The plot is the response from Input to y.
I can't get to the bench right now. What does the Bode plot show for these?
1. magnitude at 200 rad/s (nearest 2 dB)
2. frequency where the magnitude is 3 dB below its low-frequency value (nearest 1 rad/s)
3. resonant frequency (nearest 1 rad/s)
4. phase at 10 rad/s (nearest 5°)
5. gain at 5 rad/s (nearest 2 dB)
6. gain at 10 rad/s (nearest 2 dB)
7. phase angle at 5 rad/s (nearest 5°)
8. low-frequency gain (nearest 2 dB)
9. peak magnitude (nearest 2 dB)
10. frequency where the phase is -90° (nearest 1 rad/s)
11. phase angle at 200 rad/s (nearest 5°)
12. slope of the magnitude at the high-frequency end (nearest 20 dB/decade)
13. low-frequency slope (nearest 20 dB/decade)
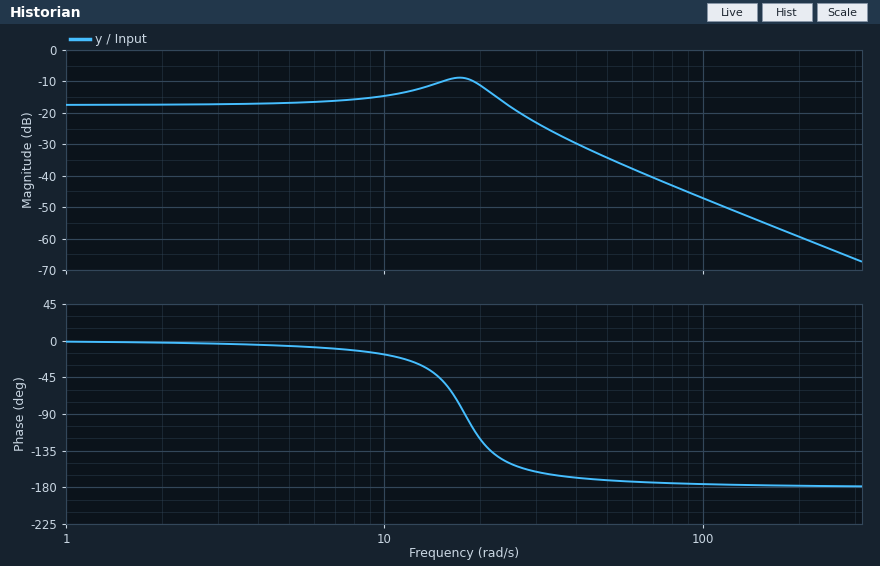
-60 dB
27 rad/s
17 rad/s
-15°
-16 dB
-14 dB
-5°
-18 dB
-8 dB
18 rad/s
-180°
-40 dB/decade
0 dB/decade
